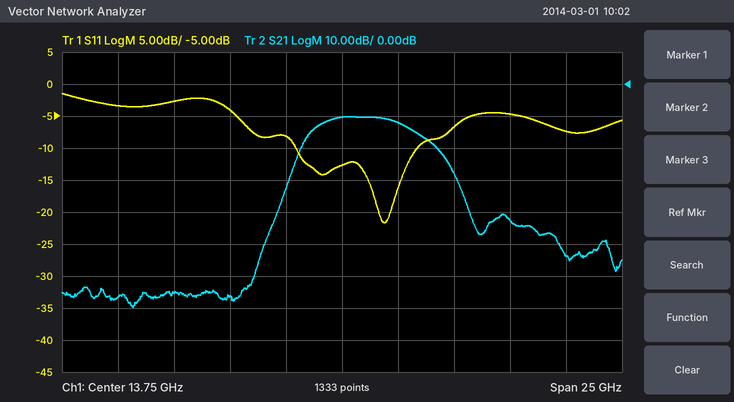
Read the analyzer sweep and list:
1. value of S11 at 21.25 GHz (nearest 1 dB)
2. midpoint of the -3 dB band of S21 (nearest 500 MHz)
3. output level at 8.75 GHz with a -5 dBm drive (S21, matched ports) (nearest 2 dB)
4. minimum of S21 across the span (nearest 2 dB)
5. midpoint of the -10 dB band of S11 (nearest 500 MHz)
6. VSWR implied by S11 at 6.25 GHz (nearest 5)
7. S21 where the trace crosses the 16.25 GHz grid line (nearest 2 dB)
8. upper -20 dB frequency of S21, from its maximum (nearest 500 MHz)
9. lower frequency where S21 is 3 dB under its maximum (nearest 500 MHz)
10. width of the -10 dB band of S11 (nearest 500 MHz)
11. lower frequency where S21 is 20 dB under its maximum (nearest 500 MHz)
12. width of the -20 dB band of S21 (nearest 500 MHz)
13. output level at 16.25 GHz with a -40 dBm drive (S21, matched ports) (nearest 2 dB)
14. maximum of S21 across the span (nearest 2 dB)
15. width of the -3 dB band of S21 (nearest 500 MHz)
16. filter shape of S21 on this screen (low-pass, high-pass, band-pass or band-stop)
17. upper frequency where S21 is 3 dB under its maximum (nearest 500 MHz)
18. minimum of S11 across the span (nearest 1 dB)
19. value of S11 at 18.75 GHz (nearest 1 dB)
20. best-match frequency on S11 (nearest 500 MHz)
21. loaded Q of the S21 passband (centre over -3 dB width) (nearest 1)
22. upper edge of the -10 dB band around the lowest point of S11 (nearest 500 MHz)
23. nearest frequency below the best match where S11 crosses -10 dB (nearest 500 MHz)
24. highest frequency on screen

-5 dB
14.5 GHz
-72 dBm
-70 dB
14.5 GHz
5
-12 dB
19.0 GHz
12.5 GHz
5.5 GHz
11.5 GHz
7.5 GHz
-52 dBm
-10 dB
4.0 GHz
band-pass
16.5 GHz
-22 dB
-7 dB
15.5 GHz
4
17.0 GHz
11.5 GHz
26.25 GHz
